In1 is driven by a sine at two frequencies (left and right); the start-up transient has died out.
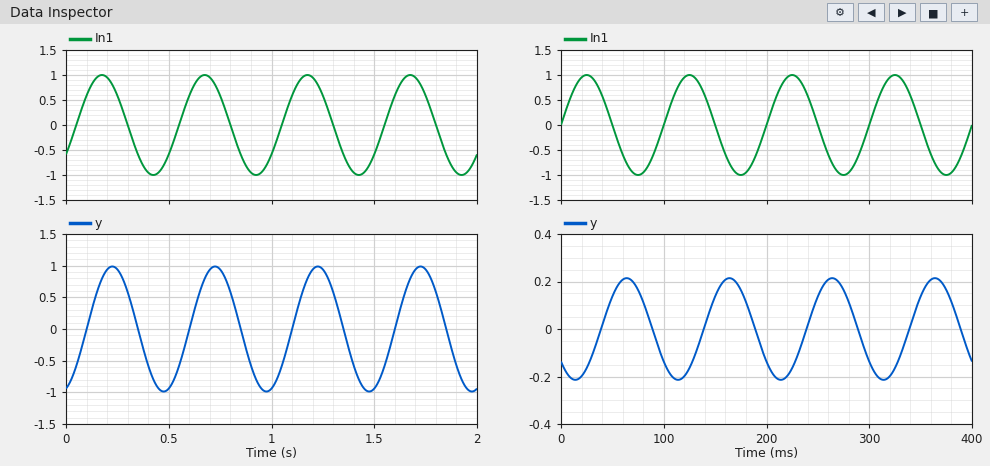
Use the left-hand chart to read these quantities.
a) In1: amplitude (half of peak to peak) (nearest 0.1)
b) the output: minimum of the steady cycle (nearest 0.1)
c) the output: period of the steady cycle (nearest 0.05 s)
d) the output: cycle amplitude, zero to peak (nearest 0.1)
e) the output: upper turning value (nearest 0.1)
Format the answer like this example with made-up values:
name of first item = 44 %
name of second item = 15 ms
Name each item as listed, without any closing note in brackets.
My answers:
In1: amplitude (half of peak to peak) = 1.0
the output: minimum of the steady cycle = -1.0
the output: period of the steady cycle = 0.50 s
the output: cycle amplitude, zero to peak = 1.0
the output: upper turning value = 1.0
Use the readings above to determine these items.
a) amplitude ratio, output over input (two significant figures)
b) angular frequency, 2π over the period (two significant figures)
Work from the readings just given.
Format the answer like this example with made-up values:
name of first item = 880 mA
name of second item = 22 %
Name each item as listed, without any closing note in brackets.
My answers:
amplitude ratio, output over input = 1.0
angular frequency, 2π over the period = 13 rad/s
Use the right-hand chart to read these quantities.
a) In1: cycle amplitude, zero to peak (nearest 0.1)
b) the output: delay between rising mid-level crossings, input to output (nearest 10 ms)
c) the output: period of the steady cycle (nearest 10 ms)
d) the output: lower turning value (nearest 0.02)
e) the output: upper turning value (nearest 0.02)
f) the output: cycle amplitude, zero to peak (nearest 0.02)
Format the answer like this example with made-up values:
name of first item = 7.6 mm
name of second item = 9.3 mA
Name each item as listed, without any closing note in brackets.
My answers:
In1: cycle amplitude, zero to peak = 1.0
the output: delay between rising mid-level crossings, input to output = 40 ms
the output: period of the steady cycle = 100 ms
the output: lower turning value = -0.22
the output: upper turning value = 0.22
the output: cycle amplitude, zero to peak = 0.22
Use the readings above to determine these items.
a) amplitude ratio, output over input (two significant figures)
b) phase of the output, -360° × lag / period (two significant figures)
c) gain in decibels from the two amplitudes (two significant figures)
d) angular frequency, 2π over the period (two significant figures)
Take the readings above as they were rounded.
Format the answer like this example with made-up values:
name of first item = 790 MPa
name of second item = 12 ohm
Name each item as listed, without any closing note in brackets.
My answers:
amplitude ratio, output over input = 0.22
phase of the output, -360° × lag / period = -140°
gain in decibels from the two amplitudes = -13 dB
angular frequency, 2π over the period = 0.063 rad/ms
